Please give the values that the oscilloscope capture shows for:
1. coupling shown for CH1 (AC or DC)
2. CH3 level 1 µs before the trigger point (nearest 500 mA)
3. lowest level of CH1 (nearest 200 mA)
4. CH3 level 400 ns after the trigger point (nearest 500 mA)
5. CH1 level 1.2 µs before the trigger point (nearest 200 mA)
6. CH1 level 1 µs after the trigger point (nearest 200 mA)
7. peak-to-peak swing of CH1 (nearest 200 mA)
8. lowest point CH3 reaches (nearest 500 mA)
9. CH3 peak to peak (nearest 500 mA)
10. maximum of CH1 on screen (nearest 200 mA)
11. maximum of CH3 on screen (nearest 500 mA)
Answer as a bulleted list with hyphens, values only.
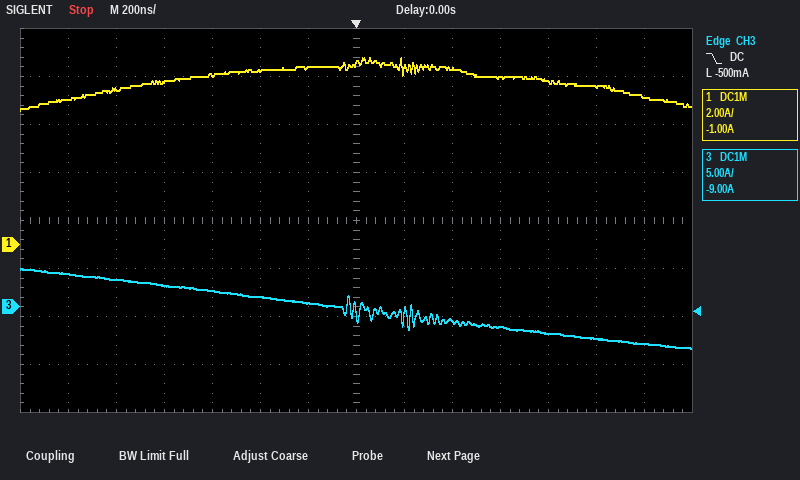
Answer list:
- DC
- 3.0 A
- 5.6 A
- -1.5 A
- 6.0 A
- 6.6 A
- 2.2 A
- -4.5 A
- 8.5 A
- 7.8 A
- 4.0 A
